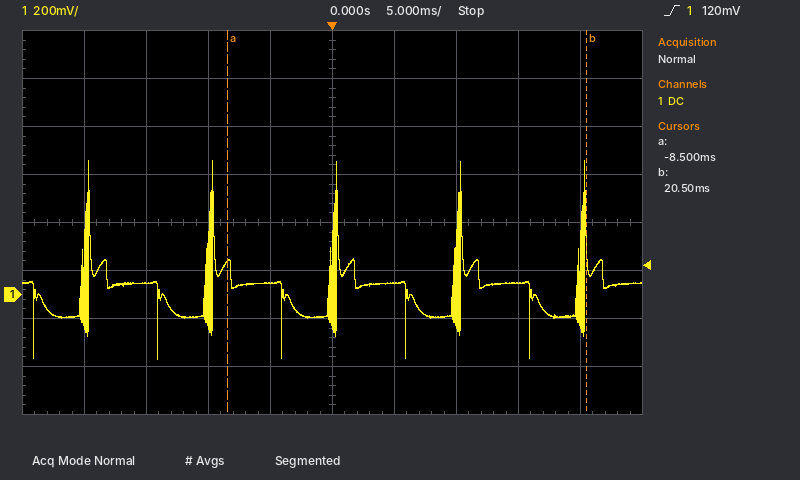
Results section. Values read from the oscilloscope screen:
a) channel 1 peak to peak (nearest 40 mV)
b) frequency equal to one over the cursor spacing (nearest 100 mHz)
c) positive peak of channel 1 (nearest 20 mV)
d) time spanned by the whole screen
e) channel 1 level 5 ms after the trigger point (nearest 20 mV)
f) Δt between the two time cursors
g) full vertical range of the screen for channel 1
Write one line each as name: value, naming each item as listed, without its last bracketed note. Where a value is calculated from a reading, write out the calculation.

channel 1 peak to peak: 840 mV
frequency equal to one over the cursor spacing: 1 / 29.0 ms ≈ 34.5 Hz
positive peak of channel 1: 560 mV
time spanned by the whole screen: 50 ms
channel 1 level 5 ms after the trigger point: 40 mV
Δt between the two time cursors: 20.5 ms − (-8.5 ms) = 29.0 ms
full vertical range of the screen for channel 1: 1.6 V
